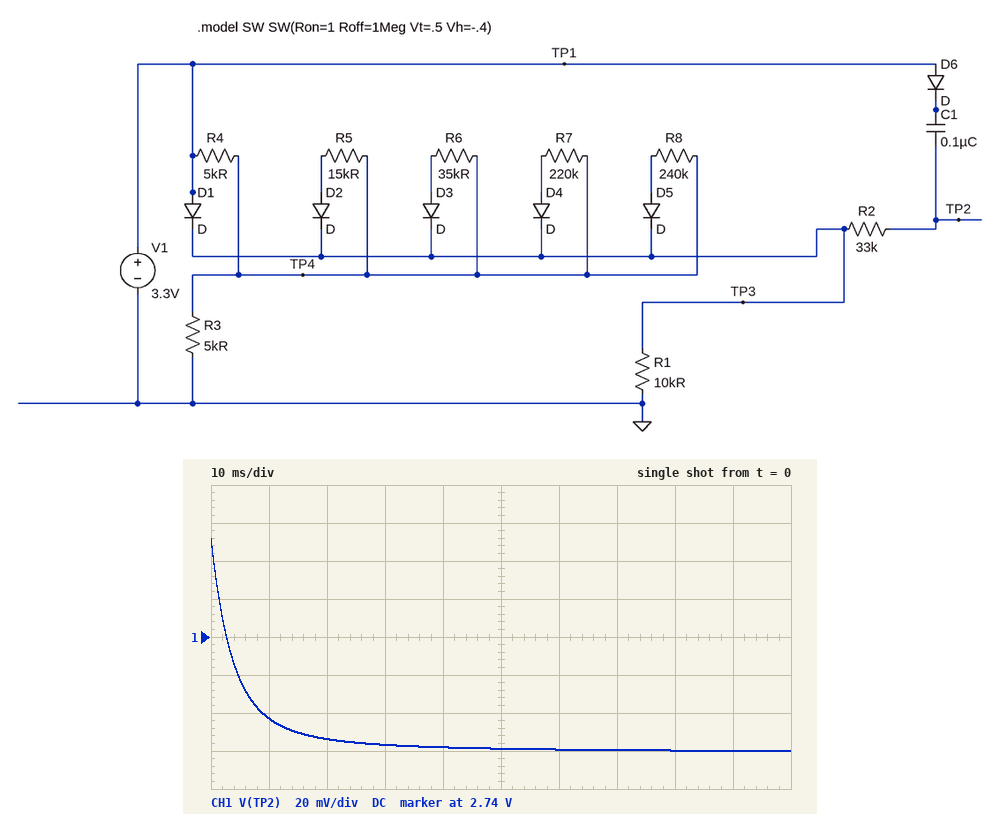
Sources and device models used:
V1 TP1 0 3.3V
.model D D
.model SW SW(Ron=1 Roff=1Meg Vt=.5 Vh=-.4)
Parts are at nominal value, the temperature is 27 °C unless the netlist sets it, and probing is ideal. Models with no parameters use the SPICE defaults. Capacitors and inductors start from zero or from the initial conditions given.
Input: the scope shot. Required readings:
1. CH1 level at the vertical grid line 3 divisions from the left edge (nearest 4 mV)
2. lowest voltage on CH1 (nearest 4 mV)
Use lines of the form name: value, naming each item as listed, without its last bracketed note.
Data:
CH1 level at the vertical grid line 3 divisions from the left edge: 2.684 V
lowest voltage on CH1: 2.680 V
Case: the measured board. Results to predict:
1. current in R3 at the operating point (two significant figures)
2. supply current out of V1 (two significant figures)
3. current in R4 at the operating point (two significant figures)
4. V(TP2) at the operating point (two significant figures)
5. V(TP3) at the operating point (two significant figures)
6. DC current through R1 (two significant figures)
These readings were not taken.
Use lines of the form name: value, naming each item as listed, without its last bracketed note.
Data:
current in R3 at the operating point: 330 µA
supply current out of V1: 600 µA
current in R4 at the operating point: 330 µA
V(TP2) at the operating point: 2.7 V
V(TP3) at the operating point: 2.7 V
DC current through R1: 270 µA
